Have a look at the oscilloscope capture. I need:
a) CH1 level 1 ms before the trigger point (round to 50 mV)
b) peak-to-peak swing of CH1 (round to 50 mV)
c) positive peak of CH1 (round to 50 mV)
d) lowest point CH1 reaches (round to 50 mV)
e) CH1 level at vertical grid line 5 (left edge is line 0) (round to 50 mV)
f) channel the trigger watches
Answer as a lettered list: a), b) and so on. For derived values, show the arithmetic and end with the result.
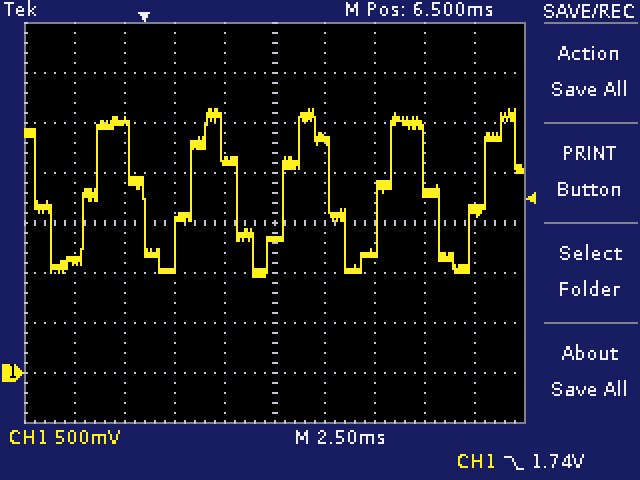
a) 2.50 V
b) 2.65 V − (950 mV) = 1.70 V
c) 2.65 V
d) 950 mV
e) 1.35 V
f) CH1
